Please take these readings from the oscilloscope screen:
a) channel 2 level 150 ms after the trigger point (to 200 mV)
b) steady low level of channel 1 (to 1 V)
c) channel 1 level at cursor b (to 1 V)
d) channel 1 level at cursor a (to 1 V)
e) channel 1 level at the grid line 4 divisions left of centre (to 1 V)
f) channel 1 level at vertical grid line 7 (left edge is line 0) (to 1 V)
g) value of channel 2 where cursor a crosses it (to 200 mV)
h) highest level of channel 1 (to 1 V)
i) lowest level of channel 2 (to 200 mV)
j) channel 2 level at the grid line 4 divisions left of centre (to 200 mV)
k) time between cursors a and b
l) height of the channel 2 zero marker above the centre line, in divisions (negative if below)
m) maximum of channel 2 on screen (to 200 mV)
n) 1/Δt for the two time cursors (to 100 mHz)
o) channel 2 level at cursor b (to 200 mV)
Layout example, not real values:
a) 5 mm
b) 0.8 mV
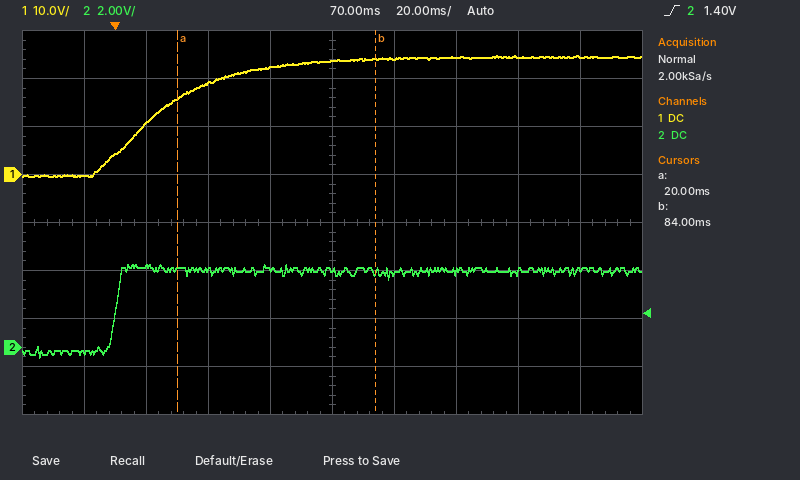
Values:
a) 3.2 V
b) 0 V
c) 24 V
d) 16 V
e) 0 V
f) 24 V
g) 3.2 V
h) 25 V
i) -400 mV
j) -200 mV
k) 64 ms
l) -2.6 div
m) 3.4 V
n) 15.6 Hz
o) 3.2 V
